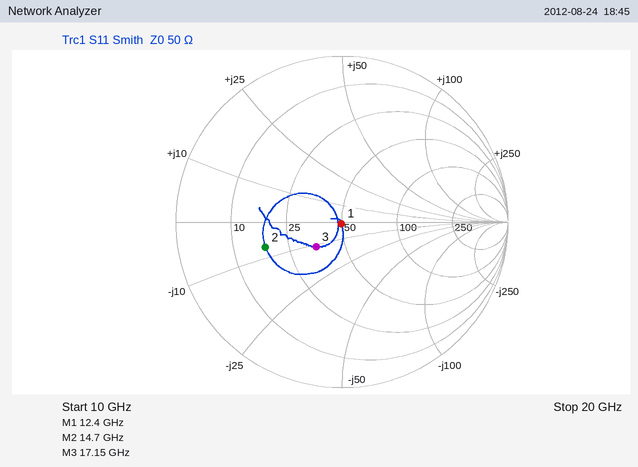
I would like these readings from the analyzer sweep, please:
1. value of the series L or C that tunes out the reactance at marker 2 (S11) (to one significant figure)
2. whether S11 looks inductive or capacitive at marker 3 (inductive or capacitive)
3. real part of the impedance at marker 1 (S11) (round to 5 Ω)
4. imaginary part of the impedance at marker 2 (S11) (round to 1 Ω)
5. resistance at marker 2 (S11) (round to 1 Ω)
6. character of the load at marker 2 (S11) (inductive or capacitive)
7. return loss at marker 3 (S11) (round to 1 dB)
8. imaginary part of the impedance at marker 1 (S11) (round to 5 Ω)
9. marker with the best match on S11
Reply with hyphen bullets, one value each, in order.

- 80 pH
- capacitive
- 50 Ω
- -7 Ω
- 18 Ω
- capacitive
- 13 dB
- 0 Ω
- marker 1
